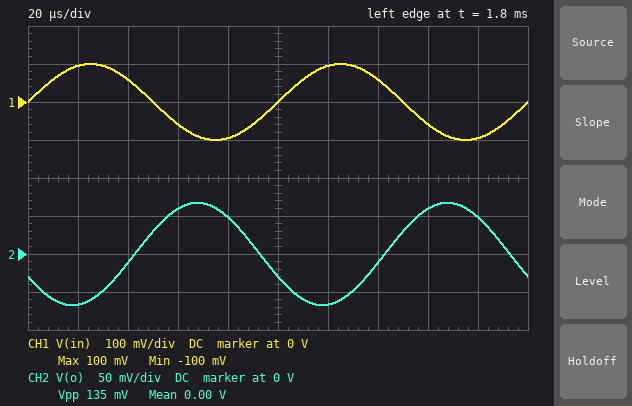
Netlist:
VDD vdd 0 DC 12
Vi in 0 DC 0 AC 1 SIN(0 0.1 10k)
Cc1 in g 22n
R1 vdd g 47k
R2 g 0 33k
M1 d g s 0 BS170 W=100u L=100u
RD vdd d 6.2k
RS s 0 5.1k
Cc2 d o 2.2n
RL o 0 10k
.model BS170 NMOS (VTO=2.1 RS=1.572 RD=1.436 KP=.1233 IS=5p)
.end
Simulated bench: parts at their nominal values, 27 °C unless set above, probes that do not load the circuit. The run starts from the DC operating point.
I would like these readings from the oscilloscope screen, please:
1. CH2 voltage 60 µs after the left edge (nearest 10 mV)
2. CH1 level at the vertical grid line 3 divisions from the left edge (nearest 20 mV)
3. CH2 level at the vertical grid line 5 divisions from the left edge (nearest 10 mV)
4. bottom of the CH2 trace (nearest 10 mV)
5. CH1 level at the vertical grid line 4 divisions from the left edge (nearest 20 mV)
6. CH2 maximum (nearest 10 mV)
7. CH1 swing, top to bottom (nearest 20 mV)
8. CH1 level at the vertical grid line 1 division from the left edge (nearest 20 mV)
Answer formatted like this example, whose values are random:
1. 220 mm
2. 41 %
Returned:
1. 60 mV
2. -60 mV
3. -30 mV
4. -70 mV
5. -100 mV
6. 70 mV
7. 200 mV
8. 100 mV
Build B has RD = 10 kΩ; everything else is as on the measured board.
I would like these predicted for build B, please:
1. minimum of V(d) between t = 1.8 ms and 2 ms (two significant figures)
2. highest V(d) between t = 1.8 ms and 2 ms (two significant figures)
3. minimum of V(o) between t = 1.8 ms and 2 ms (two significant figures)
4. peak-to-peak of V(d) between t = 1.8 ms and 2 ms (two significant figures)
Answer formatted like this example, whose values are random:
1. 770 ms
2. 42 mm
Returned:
1. 6.5 V
2. 6.7 V
3. -91 mV
4. 220 mV
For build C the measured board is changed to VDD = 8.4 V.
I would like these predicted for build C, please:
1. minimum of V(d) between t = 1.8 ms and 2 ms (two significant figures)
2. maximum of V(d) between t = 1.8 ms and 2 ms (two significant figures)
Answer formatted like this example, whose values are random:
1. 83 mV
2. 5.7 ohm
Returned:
1. 6.7 V
2. 6.9 V
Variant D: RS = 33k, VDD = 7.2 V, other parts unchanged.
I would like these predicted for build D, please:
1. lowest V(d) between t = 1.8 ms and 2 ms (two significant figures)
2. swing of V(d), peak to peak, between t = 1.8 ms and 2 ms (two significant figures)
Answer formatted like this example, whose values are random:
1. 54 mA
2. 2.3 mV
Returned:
1. 7.0 V
2. 26 mV
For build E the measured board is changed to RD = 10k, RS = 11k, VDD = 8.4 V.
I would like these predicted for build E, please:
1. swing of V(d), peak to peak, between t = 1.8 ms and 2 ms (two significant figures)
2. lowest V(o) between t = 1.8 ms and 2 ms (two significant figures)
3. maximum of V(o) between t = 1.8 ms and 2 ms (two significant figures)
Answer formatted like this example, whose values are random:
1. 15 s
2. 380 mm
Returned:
1. 100 mV
2. -42 mV
3. 42 mV
